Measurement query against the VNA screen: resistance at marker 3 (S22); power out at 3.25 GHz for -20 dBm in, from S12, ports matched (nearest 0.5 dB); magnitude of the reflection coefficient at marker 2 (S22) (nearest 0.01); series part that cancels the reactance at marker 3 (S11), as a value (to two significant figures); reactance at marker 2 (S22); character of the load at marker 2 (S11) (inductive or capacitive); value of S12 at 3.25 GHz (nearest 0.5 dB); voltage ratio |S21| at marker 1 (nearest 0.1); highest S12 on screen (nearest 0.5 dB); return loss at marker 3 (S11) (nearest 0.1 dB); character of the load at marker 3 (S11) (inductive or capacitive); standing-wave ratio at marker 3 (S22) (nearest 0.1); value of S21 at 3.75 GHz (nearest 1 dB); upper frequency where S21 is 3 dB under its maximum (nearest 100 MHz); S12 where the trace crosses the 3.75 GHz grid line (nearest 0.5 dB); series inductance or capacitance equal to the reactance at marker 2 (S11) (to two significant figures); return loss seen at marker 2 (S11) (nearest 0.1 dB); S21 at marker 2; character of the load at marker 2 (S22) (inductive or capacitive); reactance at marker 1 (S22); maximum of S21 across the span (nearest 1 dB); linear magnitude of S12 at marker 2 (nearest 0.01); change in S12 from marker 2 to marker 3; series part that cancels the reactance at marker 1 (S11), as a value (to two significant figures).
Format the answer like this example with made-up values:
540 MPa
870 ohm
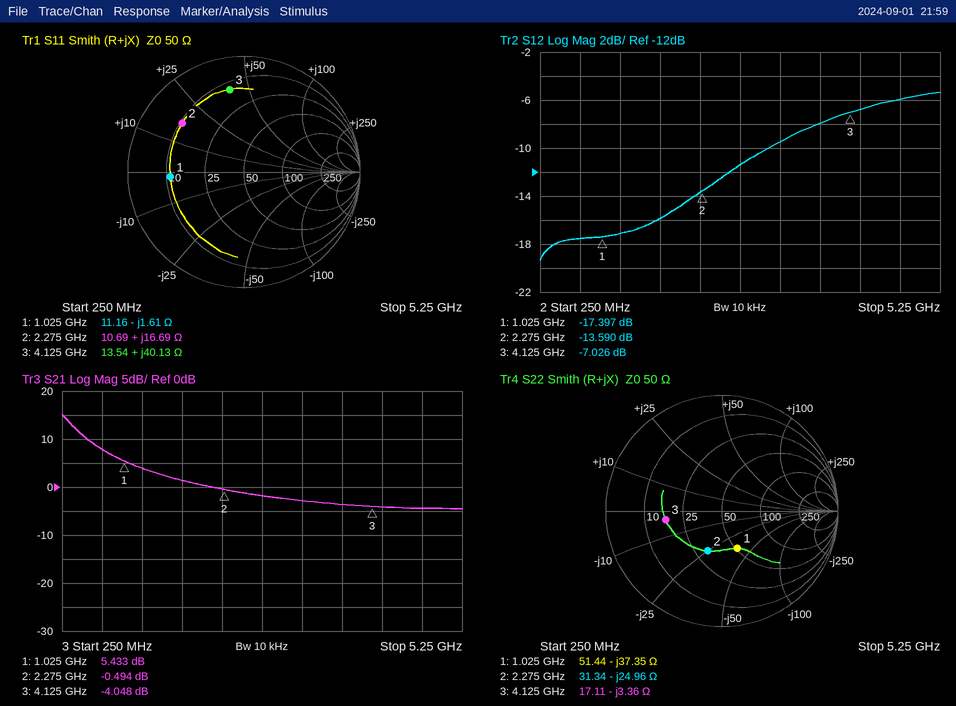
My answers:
17.11 Ω
-29.5 dBm
0.37
960 fF
-24.96 Ω
inductive
-9.5 dB
1.9
-5.5 dB
2.8 dB
inductive
2.9
-4 dB
400 MHz
-8.0 dB
1.2 nH
3.4 dB
-0.494 dB
capacitive
-37.35 Ω
15 dB
0.21
6.564 dB
250 pH
